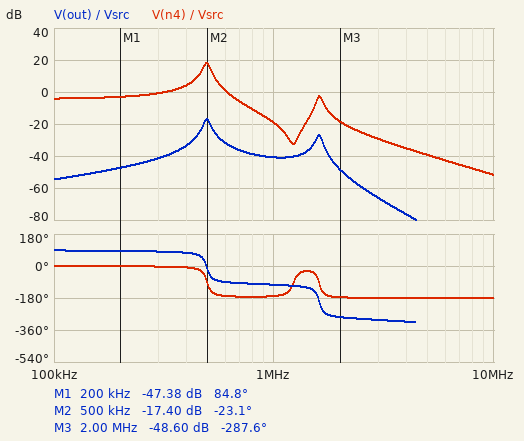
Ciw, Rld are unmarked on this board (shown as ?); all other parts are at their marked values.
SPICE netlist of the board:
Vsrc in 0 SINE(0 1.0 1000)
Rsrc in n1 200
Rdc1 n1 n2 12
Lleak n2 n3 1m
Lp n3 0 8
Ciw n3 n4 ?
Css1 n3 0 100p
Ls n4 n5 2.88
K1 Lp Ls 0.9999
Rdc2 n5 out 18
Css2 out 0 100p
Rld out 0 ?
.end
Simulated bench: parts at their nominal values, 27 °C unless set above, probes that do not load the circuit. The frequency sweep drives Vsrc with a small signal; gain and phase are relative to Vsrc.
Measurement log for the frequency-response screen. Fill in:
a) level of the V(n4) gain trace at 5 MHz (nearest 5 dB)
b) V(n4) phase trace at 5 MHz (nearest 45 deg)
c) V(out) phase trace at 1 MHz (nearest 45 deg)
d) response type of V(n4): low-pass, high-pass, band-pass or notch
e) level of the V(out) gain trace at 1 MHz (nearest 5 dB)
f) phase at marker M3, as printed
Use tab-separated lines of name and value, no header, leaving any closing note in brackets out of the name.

level of the V(n4) gain trace at 5 MHz	-40 dB
V(n4) phase trace at 5 MHz	-180 deg
V(out) phase trace at 1 MHz	-90 deg
response type of V(n4): low-pass, high-pass, band-pass or notch	low-pass
level of the V(out) gain trace at 1 MHz	-40 dB
phase at marker M3, as printed	-287.6 deg
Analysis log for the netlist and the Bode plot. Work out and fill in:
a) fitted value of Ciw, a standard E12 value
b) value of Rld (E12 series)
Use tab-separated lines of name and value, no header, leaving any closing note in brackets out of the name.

fitted value of Ciw, a standard E12 value	18 pF
value of Rld	390 Ω
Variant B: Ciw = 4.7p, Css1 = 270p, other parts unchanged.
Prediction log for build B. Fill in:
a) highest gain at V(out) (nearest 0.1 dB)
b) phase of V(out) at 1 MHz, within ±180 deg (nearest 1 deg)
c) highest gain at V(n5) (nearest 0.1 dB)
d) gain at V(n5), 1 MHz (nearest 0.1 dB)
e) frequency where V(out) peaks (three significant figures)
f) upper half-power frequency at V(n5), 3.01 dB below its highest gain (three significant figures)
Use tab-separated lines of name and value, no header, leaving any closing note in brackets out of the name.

highest gain at V(out)	-37.8 dB
phase of V(out) at 1 MHz, within ±180 deg	-102 deg
highest gain at V(n5)	-37.4 dB
gain at V(n5), 1 MHz	-65.4 dB
frequency where V(out) peaks	306 kHz
upper half-power frequency at V(n5), 3.01 dB below its highest gain	323 kHz
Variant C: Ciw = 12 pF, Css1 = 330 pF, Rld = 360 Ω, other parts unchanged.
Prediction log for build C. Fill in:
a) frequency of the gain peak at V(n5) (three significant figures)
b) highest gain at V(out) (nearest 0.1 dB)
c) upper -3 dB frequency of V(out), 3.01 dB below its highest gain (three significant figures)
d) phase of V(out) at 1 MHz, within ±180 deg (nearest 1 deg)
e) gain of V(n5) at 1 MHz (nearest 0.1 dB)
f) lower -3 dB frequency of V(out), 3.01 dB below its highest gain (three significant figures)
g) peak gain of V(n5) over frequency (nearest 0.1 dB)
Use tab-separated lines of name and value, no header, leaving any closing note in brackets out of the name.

frequency of the gain peak at V(n5)	276 kHz
highest gain at V(out)	-32.0 dB
upper -3 dB frequency of V(out), 3.01 dB below its highest gain	294 kHz
phase of V(out) at 1 MHz, within ±180 deg	-103 deg
gain of V(n5) at 1 MHz	-58.1 dB
lower -3 dB frequency of V(out), 3.01 dB below its highest gain	260 kHz
peak gain of V(n5) over frequency	-31.6 dB
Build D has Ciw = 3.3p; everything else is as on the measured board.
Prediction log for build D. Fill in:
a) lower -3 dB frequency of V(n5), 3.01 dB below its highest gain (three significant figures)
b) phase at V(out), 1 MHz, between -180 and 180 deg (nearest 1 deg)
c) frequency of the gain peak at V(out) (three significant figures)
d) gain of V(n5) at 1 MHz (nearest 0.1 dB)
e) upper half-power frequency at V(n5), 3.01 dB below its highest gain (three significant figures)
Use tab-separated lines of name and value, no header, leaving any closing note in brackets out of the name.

lower -3 dB frequency of V(n5), 3.01 dB below its highest gain	485 kHz
phase at V(out), 1 MHz, between -180 and 180 deg	-102 deg
frequency of the gain peak at V(out)	502 kHz
gain of V(n5) at 1 MHz	-58.5 dB
upper half-power frequency at V(n5), 3.01 dB below its highest gain	519 kHz
